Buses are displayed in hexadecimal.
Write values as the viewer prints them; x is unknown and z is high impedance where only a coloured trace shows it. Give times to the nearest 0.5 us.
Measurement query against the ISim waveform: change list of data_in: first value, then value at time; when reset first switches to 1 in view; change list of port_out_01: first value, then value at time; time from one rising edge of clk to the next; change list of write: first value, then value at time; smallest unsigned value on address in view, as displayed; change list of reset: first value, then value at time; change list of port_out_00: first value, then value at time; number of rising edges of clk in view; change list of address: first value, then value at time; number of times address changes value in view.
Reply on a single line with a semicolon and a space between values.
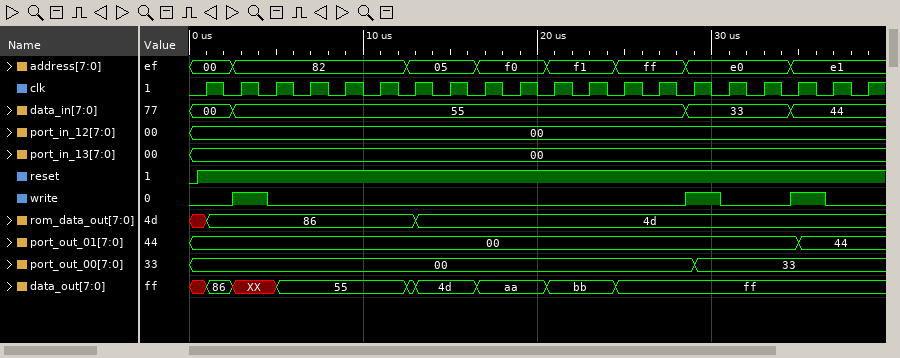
00, 55 at 2.5 us, 33 at 28.5 us, 44 at 34.5 us; 0.5 us; 00, 44 at 35 us; 2 us; 0, 1 at 2.5 us, 0 at 4.5 us, 1 at 28.5 us, 0 at 30.5 us, 1 at 34.5 us, 0 at 36.5 us; 00; 0, 1 at 0.5 us; 00, 33 at 29 us; 20; 00, 82 at 2.5 us, 05 at 12.5 us, f0 at 16.5 us, f1 at 20.5 us, ff at 24.5 us, e0 at 28.5 us, e1 at 34.5 us; 7
